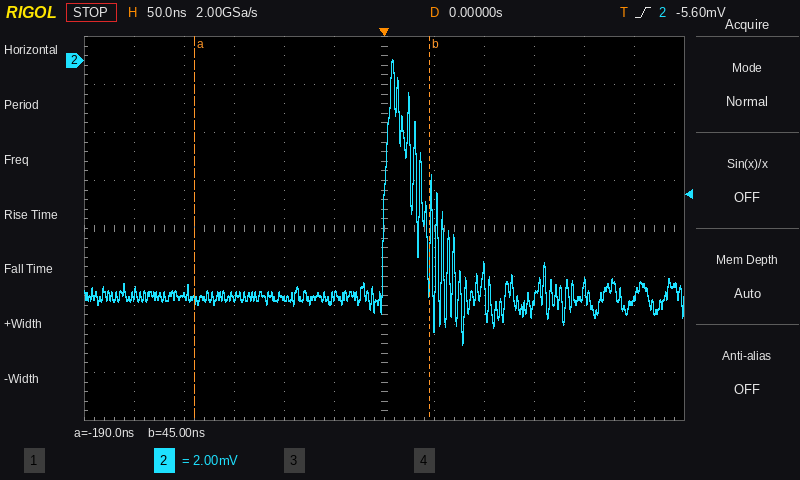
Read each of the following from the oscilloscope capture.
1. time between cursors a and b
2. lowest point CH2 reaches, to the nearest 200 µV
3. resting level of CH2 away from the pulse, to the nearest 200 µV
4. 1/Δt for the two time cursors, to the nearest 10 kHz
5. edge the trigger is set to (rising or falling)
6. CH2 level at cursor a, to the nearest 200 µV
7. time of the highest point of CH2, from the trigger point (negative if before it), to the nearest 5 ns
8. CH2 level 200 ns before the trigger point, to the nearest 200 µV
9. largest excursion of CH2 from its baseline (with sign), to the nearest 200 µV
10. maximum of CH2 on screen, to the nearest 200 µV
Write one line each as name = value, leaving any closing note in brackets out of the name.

time between cursors a and b = 235 ns
lowest point CH2 reaches, to the nearest 200 µV = -11.8 mV
resting level of CH2 away from the pulse, to the nearest 200 µV = -9.8 mV
1/Δt for the two time cursors, to the nearest 10 kHz = 4.26 MHz
edge the trigger is set to = rising
CH2 level at cursor a, to the nearest 200 µV = -10.0 mV
time of the highest point of CH2, from the trigger point (negative if before it), to the nearest 5 ns = +10 ns
CH2 level 200 ns before the trigger point, to the nearest 200 µV = -9.8 mV
largest excursion of CH2 from its baseline (with sign), to the nearest 200 µV = +9.8 mV
maximum of CH2 on screen, to the nearest 200 µV = 0.0 mV
